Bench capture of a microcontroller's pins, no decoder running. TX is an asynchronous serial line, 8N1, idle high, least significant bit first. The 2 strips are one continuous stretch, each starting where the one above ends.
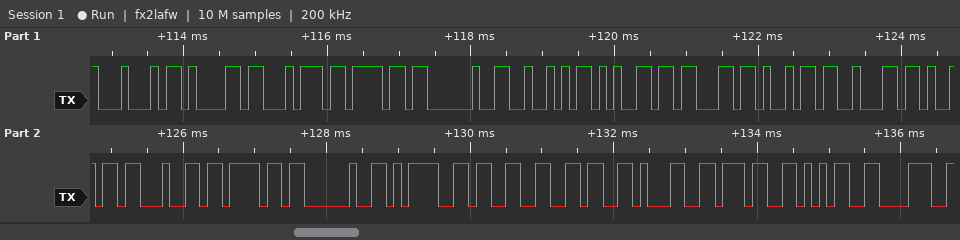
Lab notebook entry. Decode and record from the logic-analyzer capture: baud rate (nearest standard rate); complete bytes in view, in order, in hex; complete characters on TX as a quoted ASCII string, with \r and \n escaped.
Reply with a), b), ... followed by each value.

a) 9600 baud
b) 44 61 74 6F 20 52 65 63 69 62 69 64 6F 20 3D 33 36 31 37 35 38
c) "Dato Recibido =361758"
